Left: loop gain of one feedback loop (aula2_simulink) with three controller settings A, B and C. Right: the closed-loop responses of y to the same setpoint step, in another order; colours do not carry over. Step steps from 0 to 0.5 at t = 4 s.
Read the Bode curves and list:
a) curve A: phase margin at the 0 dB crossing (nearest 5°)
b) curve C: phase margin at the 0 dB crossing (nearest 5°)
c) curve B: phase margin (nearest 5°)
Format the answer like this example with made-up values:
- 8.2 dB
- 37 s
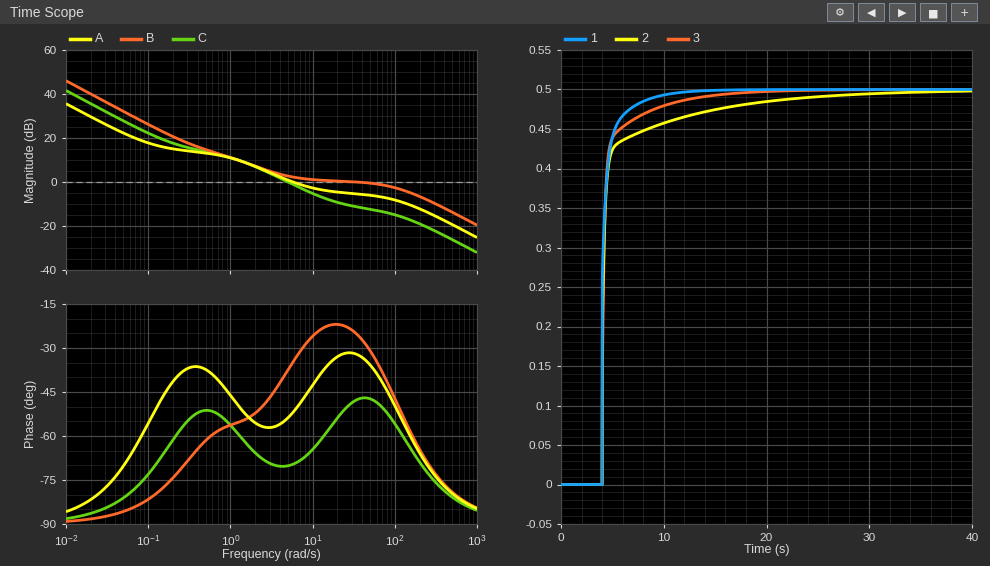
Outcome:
- 130°
- 110°
- 155°
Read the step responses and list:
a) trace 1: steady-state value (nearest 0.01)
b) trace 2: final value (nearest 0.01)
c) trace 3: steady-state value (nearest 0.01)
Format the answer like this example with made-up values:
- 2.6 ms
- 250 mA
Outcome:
- 0.50
- 0.50
- 0.50
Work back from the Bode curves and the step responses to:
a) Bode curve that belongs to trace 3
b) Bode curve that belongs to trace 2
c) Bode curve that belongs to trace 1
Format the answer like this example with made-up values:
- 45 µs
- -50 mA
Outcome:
- C
- A
- B
